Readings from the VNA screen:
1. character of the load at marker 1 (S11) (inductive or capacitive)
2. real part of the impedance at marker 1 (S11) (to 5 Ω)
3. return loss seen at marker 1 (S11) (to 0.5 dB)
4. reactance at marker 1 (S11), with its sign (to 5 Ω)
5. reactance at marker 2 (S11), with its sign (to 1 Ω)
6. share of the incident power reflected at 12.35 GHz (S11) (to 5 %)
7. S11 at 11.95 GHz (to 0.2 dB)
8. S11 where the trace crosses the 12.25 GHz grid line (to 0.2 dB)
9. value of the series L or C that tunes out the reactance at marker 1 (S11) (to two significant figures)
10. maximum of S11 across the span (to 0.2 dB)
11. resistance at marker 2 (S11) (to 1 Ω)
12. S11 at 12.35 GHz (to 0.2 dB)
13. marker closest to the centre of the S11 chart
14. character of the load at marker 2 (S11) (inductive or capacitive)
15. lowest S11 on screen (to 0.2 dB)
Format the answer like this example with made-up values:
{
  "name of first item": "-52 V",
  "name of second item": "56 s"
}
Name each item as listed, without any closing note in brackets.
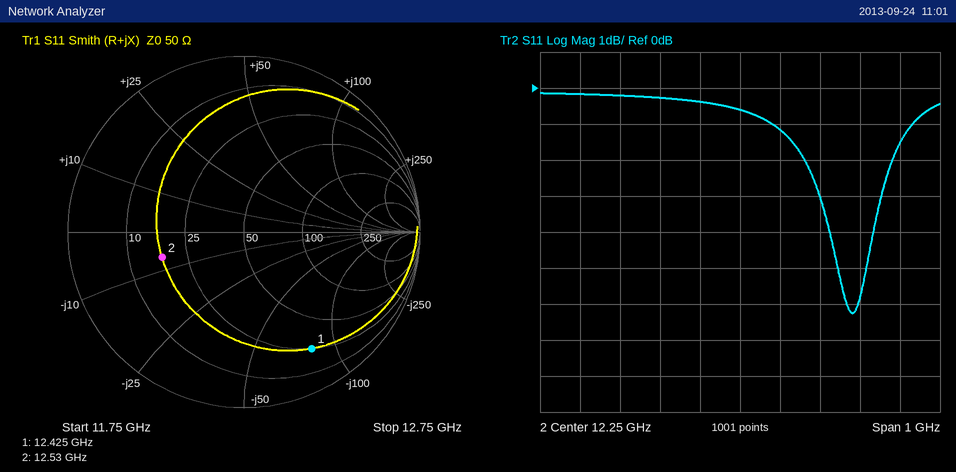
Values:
{
  "character of the load at marker 1 (S11)": "capacitive",
  "real part of the impedance at marker 1 (S11)": "25 Ω",
  "return loss seen at marker 1 (S11)": "2.5 dB",
  "reactance at marker 1 (S11), with its sign": "-80 Ω",
  "reactance at marker 2 (S11), with its sign": "-7 Ω",
  "share of the incident power reflected at 12.35 GHz (S11)": "75 %",
  "S11 at 11.95 GHz": "-0.2 dB",
  "S11 where the trace crosses the 12.25 GHz grid line": "-0.6 dB",
  "value of the series L or C that tunes out the reactance at marker 1 (S11)": "1.0 nH",
  "maximum of S11 across the span": "-0.2 dB",
  "resistance at marker 2 (S11)": "18 Ω",
  "S11 at 12.35 GHz": "-1.2 dB",
  "marker closest to the centre of the S11 chart": "marker 2",
  "character of the load at marker 2 (S11)": "capacitive",
  "lowest S11 on screen": "-6.2 dB"
}
